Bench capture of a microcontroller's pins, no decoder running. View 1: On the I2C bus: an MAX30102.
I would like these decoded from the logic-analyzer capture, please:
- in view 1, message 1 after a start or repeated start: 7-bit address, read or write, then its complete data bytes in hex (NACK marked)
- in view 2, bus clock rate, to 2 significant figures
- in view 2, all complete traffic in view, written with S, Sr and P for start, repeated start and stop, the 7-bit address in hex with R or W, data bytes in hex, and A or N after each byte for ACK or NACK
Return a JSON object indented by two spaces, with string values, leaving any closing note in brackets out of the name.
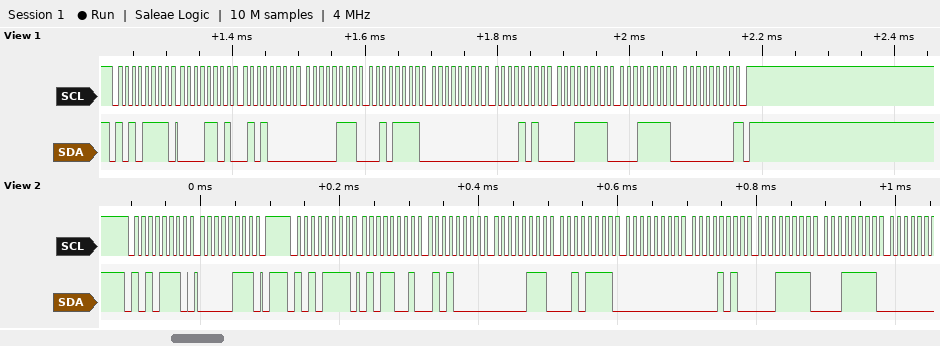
{
  "in view 1, message 1 after a start or repeated start: 7-bit address, read or write, then its complete data bytes in hex": "0x57 read: 0D 50 07 2F 00 0A 1F 1F 00 NACK",
  "in view 2, bus clock rate, to 2 significant figures": "100 kHz",
  "in view 2, all complete traffic in view, written with S, Sr and P for start, repeated start and stop, the 7-bit address in hex with R or W, data bytes in hex, and A or N after each byte for ACK or NACK": "S 57W A 07 A P S 57R A 59 A 50 A 07 A 2F A 00 A 0A A 1F A 1F A"
}
